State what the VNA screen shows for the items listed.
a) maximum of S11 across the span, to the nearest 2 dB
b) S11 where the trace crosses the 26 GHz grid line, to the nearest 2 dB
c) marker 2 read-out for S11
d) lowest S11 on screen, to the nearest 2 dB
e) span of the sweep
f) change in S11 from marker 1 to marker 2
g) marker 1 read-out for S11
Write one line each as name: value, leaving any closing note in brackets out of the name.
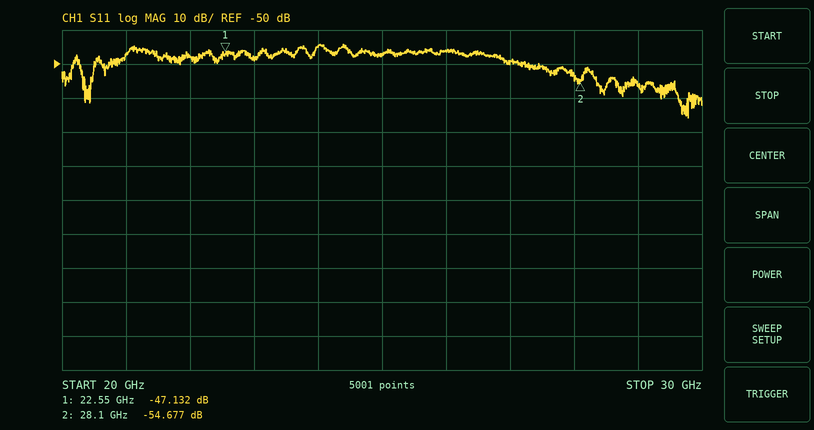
maximum of S11 across the span, to the nearest 2 dB: -44 dB
S11 where the trace crosses the 26 GHz grid line, to the nearest 2 dB: -46 dB
marker 2 read-out for S11: -54.677 dB
lowest S11 on screen, to the nearest 2 dB: -66 dB
span of the sweep: 10 GHz
change in S11 from marker 1 to marker 2: -7.545 dB
marker 1 read-out for S11: -47.132 dB
